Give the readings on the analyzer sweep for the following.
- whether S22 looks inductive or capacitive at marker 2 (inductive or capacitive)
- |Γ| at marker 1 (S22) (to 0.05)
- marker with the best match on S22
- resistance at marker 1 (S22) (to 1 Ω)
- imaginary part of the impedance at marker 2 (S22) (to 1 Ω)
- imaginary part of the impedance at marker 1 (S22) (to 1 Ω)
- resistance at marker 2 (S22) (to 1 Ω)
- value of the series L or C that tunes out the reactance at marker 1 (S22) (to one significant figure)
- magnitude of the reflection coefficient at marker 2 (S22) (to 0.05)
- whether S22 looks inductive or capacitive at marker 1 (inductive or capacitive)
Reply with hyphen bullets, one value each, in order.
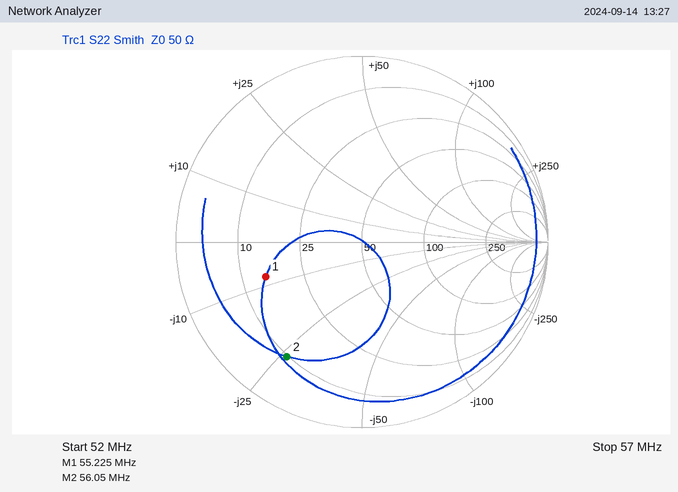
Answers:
- capacitive
- 0.55
- marker 1
- 15 Ω
- -26 Ω
- -8 Ω
- 10 Ω
- 20 nH
- 0.75
- capacitive
